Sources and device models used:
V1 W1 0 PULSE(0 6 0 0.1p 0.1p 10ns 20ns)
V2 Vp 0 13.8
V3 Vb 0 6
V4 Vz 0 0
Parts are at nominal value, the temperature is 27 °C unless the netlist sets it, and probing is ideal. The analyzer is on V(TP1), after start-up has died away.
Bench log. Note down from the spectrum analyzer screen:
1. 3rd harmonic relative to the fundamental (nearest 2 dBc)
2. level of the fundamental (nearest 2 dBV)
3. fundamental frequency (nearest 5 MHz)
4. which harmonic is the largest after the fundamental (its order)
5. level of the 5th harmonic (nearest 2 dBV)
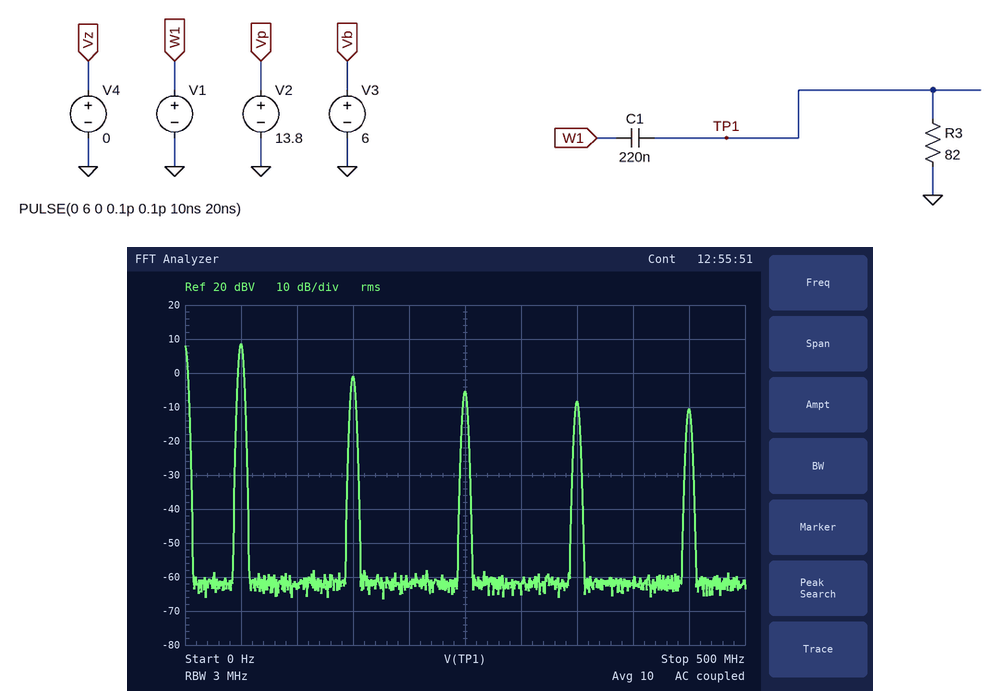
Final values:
-10 dBc
8 dBV
50 MHz
3
-6 dBV
